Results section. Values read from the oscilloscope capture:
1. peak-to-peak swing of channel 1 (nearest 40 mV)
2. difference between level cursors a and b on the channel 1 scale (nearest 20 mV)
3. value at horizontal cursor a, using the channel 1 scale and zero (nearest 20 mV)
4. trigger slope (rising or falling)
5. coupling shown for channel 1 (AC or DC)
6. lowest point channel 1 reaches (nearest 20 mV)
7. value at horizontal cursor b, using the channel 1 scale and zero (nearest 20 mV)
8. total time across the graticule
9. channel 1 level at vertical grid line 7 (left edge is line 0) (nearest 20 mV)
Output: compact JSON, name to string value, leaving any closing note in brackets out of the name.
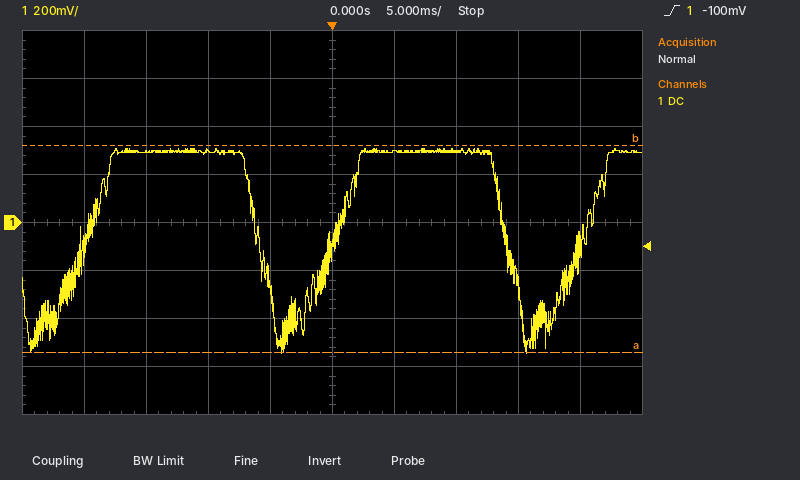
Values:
{"peak-to-peak swing of channel 1": "840 mV", "difference between level cursors a and b on the channel 1 scale": "860 mV", "value at horizontal cursor a, using the channel 1 scale and zero": "-540 mV", "trigger slope": "rising", "coupling shown for channel 1": "DC", "lowest point channel 1 reaches": "-540 mV", "value at horizontal cursor b, using the channel 1 scale and zero": "320 mV", "total time across the graticule": "50 ms", "channel 1 level at vertical grid line 7 (left edge is line 0)": "300 mV"}
